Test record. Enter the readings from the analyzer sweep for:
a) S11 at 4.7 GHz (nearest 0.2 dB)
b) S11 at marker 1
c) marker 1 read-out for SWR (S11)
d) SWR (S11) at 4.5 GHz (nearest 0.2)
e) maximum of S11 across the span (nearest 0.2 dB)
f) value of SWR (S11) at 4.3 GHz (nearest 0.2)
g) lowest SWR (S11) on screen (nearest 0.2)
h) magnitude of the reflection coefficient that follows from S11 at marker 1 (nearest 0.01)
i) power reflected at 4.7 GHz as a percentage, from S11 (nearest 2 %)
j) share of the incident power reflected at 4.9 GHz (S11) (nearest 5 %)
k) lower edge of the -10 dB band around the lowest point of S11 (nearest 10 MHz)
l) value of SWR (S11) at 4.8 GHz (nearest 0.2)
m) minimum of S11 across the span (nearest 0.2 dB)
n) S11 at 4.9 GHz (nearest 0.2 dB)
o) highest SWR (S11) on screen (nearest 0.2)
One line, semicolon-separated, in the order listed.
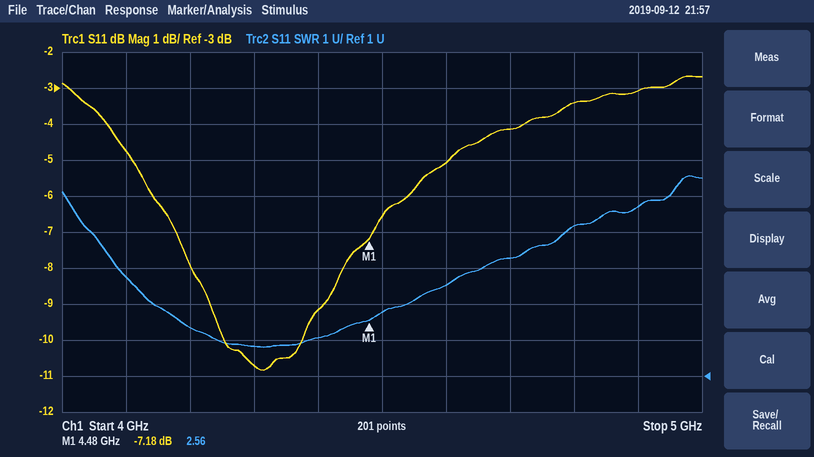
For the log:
-4.2 dB; -7.18 dB; 2.56; 2.8; -2.6 dB; 1.8; 1.8; 0.44; 38 %; 50 %; 4.25 GHz; 5.2; -10.8 dB; -3.0 dB; 6.6
